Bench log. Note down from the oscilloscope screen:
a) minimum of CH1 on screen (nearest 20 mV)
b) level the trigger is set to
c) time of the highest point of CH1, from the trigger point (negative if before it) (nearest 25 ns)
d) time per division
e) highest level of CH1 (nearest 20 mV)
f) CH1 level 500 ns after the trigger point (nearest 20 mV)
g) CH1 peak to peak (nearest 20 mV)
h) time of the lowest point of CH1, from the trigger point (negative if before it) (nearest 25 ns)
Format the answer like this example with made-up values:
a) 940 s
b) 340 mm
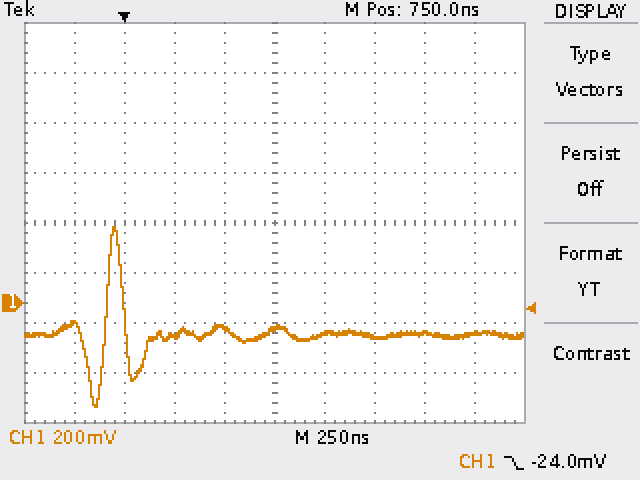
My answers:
a) -420 mV
b) -24.0 mV
c) -50 ns
d) 250 ns
e) 300 mV
f) -100 mV
g) 720 mV
h) -150 ns
